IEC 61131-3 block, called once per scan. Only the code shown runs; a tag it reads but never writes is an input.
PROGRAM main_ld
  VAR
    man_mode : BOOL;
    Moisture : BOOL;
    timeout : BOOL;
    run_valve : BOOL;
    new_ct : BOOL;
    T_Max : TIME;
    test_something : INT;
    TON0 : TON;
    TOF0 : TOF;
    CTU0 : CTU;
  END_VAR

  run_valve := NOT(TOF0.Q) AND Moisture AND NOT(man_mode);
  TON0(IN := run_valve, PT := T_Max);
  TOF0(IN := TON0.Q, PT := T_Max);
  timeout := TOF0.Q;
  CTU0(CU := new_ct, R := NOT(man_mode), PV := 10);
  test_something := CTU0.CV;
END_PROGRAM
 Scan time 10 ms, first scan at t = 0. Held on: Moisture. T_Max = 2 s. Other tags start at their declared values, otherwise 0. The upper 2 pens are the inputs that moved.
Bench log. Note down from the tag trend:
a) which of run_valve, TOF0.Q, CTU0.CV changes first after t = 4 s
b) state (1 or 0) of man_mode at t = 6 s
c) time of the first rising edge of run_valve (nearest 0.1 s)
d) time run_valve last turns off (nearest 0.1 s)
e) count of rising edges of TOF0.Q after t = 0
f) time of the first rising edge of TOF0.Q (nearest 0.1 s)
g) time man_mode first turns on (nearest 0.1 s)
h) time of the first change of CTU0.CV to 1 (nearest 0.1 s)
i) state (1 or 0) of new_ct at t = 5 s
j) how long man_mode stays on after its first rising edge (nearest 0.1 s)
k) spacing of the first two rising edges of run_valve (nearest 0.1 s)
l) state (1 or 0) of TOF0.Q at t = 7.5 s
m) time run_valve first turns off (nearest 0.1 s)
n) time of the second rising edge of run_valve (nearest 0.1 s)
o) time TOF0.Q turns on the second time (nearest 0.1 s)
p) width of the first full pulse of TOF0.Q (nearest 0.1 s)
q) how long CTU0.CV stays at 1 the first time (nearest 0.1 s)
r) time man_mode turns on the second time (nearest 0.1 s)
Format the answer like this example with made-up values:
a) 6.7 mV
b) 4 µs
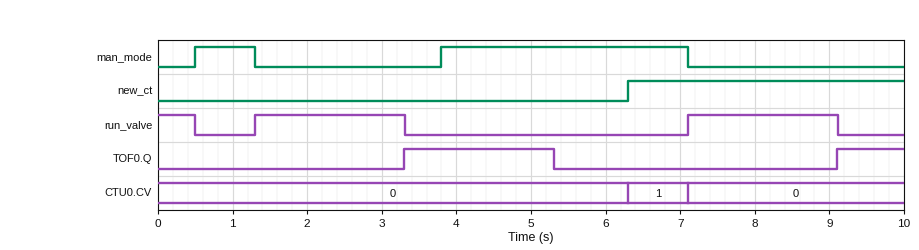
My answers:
a) TOF0.Q
b) 1
c) 1.3 s
d) 9.1 s
e) 2
f) 3.3 s
g) 0.5 s
h) 6.3 s
i) 0
j) 0.8 s
k) 5.8 s
l) 0
m) 0.5 s
n) 7.1 s
o) 9.1 s
p) 2.0 s
q) 0.8 s
r) 3.8 s
